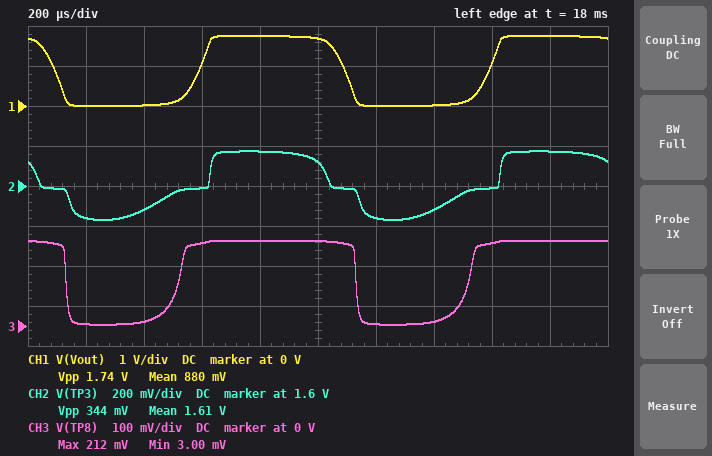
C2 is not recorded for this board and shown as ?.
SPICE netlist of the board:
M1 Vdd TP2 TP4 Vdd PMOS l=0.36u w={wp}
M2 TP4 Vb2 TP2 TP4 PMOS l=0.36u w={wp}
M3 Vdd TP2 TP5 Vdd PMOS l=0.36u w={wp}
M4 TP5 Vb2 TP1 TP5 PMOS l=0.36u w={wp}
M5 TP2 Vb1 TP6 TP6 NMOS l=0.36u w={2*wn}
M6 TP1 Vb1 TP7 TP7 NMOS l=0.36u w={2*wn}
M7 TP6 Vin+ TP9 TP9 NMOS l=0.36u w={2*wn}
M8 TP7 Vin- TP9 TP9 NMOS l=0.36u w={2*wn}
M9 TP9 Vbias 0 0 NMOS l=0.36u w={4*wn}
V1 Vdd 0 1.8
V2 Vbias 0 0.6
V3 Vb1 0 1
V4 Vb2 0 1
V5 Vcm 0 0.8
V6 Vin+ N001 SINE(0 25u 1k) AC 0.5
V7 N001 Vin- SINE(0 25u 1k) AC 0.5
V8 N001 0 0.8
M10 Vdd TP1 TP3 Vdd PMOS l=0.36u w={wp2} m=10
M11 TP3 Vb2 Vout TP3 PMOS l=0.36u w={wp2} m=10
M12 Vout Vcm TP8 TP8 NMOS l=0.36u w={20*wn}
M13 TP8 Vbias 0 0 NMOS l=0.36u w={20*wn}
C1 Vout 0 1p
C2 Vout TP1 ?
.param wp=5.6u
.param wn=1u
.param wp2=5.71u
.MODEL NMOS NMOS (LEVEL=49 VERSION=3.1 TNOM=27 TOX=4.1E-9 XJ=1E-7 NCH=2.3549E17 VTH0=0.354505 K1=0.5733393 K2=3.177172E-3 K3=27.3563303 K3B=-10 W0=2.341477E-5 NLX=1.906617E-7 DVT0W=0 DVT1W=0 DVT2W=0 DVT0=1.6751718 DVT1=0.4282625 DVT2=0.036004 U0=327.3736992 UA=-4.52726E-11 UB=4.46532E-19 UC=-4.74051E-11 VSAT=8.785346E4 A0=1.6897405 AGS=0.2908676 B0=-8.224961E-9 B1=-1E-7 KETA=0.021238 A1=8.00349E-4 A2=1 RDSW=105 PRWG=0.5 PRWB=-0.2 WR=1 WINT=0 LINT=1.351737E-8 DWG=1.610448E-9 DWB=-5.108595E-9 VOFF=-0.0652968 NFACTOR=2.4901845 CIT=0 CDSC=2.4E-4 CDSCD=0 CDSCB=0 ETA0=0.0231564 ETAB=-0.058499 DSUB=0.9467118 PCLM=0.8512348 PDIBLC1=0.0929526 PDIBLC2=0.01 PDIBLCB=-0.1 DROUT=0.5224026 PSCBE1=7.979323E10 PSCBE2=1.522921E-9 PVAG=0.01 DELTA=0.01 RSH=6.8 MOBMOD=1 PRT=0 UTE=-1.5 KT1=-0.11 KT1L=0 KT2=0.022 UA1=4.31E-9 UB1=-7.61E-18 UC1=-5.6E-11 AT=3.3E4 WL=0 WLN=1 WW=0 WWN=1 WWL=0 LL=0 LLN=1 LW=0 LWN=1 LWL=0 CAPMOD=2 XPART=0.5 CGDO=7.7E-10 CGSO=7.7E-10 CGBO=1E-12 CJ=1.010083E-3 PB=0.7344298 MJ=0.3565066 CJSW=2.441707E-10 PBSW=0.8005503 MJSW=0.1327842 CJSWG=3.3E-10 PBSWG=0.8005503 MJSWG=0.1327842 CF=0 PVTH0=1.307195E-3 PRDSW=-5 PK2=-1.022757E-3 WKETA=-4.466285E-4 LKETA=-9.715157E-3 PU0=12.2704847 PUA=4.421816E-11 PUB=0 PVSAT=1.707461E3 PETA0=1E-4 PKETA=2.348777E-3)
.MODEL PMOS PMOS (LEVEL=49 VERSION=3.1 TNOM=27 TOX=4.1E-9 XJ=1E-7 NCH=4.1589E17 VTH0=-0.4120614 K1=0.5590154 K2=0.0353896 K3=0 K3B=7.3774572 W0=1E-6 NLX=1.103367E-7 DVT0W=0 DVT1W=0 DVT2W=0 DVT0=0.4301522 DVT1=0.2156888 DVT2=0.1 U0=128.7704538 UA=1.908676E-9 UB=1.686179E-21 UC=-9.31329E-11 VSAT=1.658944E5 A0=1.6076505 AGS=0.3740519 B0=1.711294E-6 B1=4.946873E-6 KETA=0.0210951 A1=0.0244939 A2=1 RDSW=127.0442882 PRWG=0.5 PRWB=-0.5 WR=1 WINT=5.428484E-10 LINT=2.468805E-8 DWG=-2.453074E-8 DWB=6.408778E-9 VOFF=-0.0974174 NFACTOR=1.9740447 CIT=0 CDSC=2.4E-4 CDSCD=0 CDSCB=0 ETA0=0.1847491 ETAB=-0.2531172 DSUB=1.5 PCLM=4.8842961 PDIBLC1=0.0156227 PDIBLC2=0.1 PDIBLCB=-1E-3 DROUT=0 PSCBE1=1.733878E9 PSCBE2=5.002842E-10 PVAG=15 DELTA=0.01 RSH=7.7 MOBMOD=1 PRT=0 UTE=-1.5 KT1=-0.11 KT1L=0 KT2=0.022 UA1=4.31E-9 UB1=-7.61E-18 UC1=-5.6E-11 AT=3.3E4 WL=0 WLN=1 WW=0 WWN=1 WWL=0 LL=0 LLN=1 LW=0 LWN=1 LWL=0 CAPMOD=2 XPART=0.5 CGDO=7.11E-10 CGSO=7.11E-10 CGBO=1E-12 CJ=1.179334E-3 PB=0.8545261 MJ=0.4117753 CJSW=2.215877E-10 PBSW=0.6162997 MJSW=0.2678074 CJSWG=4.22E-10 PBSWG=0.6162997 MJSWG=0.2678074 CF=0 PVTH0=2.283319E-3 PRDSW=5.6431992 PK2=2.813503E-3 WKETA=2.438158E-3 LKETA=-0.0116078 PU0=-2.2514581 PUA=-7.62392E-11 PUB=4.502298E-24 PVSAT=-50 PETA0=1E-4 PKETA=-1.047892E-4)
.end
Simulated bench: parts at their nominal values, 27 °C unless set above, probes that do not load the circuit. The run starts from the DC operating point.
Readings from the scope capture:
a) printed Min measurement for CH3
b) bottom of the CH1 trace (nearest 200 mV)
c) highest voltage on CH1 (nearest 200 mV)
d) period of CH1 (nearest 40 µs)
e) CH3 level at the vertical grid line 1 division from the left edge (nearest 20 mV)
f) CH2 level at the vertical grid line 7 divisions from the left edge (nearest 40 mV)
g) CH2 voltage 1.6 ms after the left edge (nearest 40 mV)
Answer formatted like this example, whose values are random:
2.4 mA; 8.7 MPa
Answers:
3.00 mV; 0 V; 1.8 V; 1.00 ms; 0 V; 1.48 V; 1.60 V
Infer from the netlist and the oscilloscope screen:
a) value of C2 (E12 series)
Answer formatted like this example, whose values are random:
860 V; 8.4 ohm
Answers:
220 fF
